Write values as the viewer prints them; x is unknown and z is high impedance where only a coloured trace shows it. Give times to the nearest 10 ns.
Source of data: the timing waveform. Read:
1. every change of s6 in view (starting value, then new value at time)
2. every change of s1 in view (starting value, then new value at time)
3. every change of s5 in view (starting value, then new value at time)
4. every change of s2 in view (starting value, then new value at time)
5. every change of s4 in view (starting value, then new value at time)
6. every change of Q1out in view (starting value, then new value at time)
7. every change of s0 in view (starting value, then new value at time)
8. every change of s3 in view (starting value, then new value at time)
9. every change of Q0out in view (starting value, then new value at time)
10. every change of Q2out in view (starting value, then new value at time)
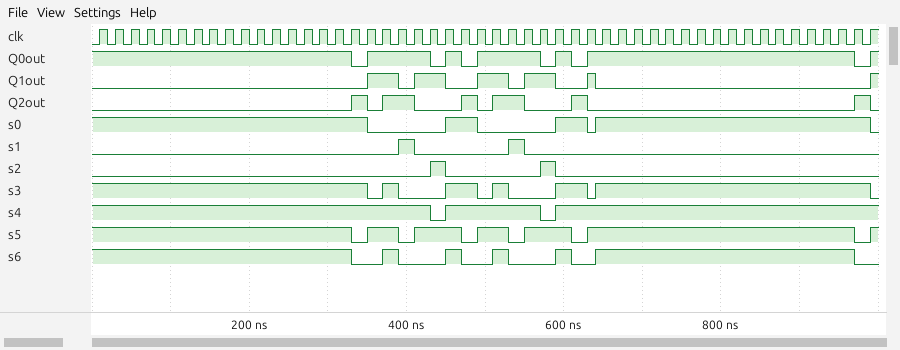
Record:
1, 0 at 330 ns, 1 at 370 ns, 0 at 390 ns, 1 at 450 ns, 0 at 470 ns, 1 at 510 ns, 0 at 530 ns, 1 at 590 ns, 0 at 610 ns, 1 at 640 ns, 0 at 970 ns
0, 1 at 390 ns, 0 at 410 ns, 1 at 530 ns, 0 at 550 ns
1, 0 at 330 ns, 1 at 350 ns, 0 at 390 ns, 1 at 410 ns, 0 at 470 ns, 1 at 490 ns, 0 at 530 ns, 1 at 550 ns, 0 at 610 ns, 1 at 630 ns, 0 at 970 ns, 1 at 990 ns
0, 1 at 430 ns, 0 at 450 ns, 1 at 570 ns, 0 at 590 ns
1, 0 at 430 ns, 1 at 450 ns, 0 at 570 ns, 1 at 590 ns
0, 1 at 350 ns, 0 at 390 ns, 1 at 410 ns, 0 at 450 ns, 1 at 490 ns, 0 at 530 ns, 1 at 550 ns, 0 at 590 ns, 1 at 630 ns, 0 at 640 ns, 1 at 990 ns
1, 0 at 350 ns, 1 at 450 ns, 0 at 490 ns, 1 at 590 ns, 0 at 630 ns, 1 at 640 ns, 0 at 990 ns
1, 0 at 350 ns, 1 at 370 ns, 0 at 390 ns, 1 at 450 ns, 0 at 490 ns, 1 at 510 ns, 0 at 530 ns, 1 at 590 ns, 0 at 630 ns, 1 at 640 ns, 0 at 990 ns
1, 0 at 330 ns, 1 at 350 ns, 0 at 430 ns, 1 at 450 ns, 0 at 470 ns, 1 at 490 ns, 0 at 570 ns, 1 at 590 ns, 0 at 610 ns, 1 at 630 ns, 0 at 970 ns, 1 at 990 ns
0, 1 at 330 ns, 0 at 350 ns, 1 at 370 ns, 0 at 410 ns, 1 at 470 ns, 0 at 490 ns, 1 at 510 ns, 0 at 550 ns, 1 at 610 ns, 0 at 630 ns, 1 at 970 ns, 0 at 990 ns
